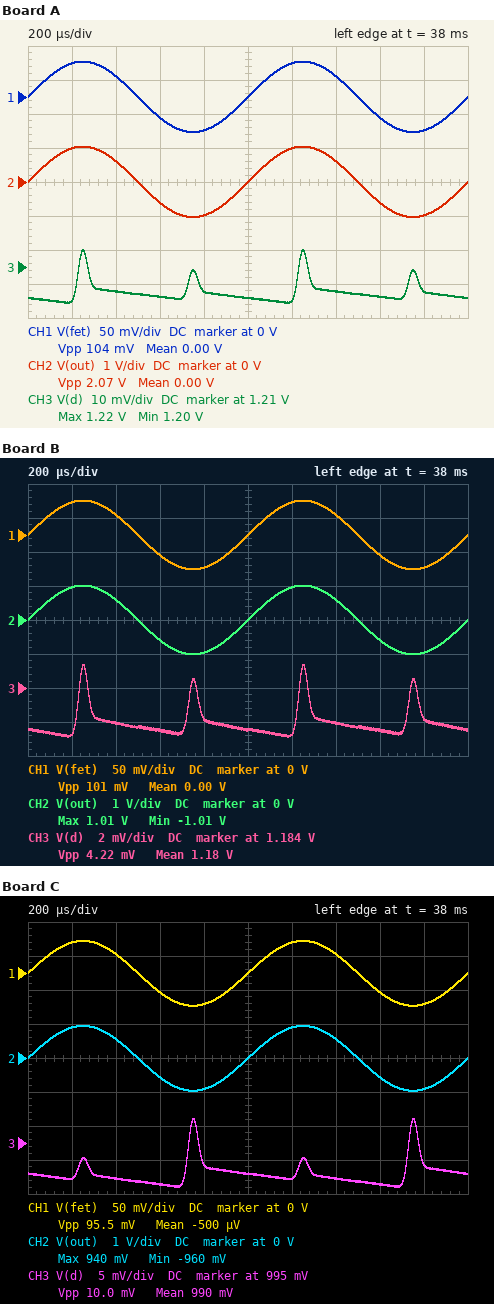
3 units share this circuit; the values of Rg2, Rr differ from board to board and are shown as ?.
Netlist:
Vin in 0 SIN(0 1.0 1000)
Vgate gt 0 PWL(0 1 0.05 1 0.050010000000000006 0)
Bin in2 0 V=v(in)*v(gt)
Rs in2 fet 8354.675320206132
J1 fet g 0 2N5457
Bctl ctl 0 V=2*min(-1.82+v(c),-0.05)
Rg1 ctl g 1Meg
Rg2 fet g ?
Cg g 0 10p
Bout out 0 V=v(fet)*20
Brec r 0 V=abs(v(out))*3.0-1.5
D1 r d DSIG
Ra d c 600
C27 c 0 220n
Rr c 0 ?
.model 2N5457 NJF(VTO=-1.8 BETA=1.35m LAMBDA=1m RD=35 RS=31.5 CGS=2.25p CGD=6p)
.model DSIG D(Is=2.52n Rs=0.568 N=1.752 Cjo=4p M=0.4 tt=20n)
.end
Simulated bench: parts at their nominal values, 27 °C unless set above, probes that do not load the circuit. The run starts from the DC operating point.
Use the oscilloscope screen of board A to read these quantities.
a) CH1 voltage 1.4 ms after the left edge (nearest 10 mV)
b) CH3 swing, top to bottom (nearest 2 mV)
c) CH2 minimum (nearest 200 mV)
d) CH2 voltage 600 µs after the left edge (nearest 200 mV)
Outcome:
30 mV
16 mV
-1.0 V
-600 mV
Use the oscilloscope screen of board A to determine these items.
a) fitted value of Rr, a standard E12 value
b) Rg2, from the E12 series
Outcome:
680 kΩ
2.2 MΩ
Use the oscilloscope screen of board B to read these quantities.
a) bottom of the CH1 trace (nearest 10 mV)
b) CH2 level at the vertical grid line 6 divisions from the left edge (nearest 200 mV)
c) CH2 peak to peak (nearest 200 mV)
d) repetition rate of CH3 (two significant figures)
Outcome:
-50 mV
1.0 V
2.0 V
2.0 kHz
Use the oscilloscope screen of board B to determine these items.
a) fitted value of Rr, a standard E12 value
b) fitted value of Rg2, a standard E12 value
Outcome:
2.2 MΩ
1.8 MΩ
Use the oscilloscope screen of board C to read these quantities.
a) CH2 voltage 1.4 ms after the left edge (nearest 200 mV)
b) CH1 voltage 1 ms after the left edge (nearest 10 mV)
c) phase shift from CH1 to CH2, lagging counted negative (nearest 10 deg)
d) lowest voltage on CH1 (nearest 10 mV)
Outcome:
600 mV
0 V
0 deg
-50 mV
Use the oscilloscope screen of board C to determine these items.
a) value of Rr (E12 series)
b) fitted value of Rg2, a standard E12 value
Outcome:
1 MΩ
820 kΩ
